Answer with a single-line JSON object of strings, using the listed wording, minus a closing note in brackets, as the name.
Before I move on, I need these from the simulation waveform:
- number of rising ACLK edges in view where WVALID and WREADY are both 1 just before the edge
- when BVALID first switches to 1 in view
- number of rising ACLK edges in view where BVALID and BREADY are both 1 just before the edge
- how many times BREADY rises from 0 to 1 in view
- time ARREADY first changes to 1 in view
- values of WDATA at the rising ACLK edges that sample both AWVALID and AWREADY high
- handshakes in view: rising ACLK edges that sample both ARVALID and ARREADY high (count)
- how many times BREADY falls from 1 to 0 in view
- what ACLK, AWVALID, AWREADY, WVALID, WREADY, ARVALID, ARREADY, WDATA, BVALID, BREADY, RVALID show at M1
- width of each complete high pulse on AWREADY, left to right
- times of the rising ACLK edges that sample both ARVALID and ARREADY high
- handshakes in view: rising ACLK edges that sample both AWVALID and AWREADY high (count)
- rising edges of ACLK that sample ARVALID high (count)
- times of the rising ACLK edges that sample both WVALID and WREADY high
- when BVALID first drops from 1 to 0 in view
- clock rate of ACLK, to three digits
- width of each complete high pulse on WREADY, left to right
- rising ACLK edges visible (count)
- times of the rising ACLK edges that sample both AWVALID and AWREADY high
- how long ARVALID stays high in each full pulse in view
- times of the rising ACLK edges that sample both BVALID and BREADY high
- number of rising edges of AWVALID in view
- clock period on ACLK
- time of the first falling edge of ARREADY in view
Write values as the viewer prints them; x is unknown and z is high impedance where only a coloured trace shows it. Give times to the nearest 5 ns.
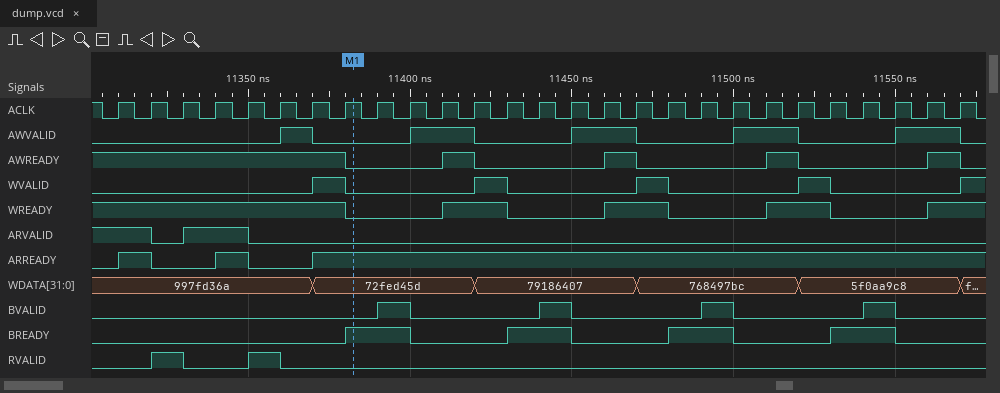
{"number of rising ACLK edges in view where WVALID and WREADY are both 1 just before the edge": "4", "when BVALID first switches to 1 in view": "11390 ns", "number of rising ACLK edges in view where BVALID and BREADY are both 1 just before the edge": "4", "how many times BREADY rises from 0 to 1 in view": "4", "time ARREADY first changes to 1 in view": "11310 ns", "values of WDATA at the rising ACLK edges that sample both AWVALID and AWREADY high": "997fd36a, 72fed45d, 79186407, 768497bc, 5f0aa9c8", "handshakes in view: rising ACLK edges that sample both ARVALID and ARREADY high": "2", "how many times BREADY falls from 1 to 0 in view": "4", "what ACLK, AWVALID, AWREADY, WVALID, WREADY, ARVALID, ARREADY, WDATA, BVALID, BREADY, RVALID show at M1": "ACLK=1, AWVALID=0, AWREADY=0, WVALID=0, WREADY=0, ARVALID=0, ARREADY=1, WDATA=72fed45d, BVALID=0, BREADY=1, RVALID=0", "width of each complete high pulse on AWREADY, left to right": "10 ns, 10 ns, 10 ns, 10 ns", "times of the rising ACLK edges that sample both ARVALID and ARREADY high": "11320 ns, 11350 ns", "handshakes in view: rising ACLK edges that sample both AWVALID and AWREADY high": "5", "rising edges of ACLK that sample ARVALID high": "4", "times of the rising ACLK edges that sample both WVALID and WREADY high": "11380 ns, 11430 ns, 11480 ns, 11530 ns", "when BVALID first drops from 1 to 0 in view": "11400 ns", "clock rate of ACLK, to three digits": "100 MHz", "width of each complete high pulse on WREADY, left to right": "20 ns, 20 ns, 20 ns", "rising ACLK edges visible": "27", "times of the rising ACLK edges that sample both AWVALID and AWREADY high": "11370 ns, 11420 ns, 11470 ns, 11520 ns, 11570 ns", "how long ARVALID stays high in each full pulse in view": "20 ns", "times of the rising ACLK edges that sample both BVALID and BREADY high": "11400 ns, 11450 ns, 11500 ns, 11550 ns", "number of rising edges of AWVALID in view": "5", "clock period on ACLK": "10 ns", "time of the first falling edge of ARREADY in view": "11320 ns"}
